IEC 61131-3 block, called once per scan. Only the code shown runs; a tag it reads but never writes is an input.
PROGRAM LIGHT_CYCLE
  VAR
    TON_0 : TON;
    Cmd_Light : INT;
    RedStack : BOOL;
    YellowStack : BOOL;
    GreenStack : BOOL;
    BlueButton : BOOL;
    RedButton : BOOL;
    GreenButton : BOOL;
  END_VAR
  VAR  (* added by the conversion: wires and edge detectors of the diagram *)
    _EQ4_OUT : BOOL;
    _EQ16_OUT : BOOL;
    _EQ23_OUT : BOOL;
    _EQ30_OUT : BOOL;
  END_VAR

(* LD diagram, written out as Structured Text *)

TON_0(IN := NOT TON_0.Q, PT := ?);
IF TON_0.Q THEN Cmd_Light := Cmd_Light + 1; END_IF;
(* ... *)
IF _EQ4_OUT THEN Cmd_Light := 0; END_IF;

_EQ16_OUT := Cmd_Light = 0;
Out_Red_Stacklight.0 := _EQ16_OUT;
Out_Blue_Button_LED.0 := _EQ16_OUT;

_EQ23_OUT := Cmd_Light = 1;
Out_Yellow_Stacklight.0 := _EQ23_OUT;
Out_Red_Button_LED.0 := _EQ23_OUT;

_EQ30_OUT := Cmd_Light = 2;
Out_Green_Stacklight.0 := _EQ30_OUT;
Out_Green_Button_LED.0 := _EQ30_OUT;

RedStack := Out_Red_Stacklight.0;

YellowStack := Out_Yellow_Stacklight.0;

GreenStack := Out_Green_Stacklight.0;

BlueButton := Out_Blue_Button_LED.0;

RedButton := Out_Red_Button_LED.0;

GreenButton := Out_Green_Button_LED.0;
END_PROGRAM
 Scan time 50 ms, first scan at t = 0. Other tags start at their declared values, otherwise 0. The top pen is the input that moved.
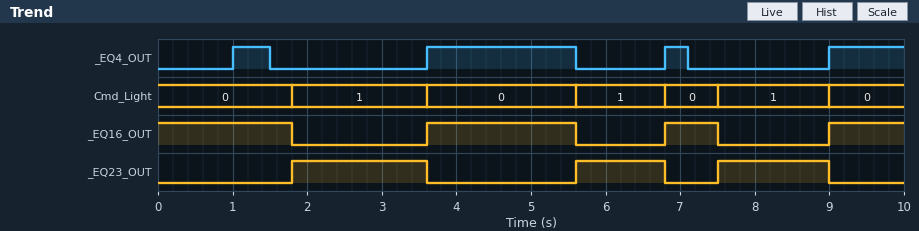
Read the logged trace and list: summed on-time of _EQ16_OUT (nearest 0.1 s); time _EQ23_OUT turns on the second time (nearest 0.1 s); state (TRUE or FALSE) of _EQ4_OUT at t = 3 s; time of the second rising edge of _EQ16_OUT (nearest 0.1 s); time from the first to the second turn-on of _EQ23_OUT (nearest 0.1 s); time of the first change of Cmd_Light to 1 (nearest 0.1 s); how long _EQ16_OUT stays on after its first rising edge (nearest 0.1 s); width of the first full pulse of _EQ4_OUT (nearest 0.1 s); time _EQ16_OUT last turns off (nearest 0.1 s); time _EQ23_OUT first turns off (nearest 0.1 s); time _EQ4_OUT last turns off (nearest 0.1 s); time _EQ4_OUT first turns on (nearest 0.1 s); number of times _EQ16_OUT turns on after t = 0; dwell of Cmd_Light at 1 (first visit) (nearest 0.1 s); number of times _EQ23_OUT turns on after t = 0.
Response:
5.5 s
5.6 s
FALSE
6.8 s
3.8 s
1.8 s
2.0 s
0.5 s
7.5 s
3.6 s
7.1 s
1.0 s
3
1.8 s
3
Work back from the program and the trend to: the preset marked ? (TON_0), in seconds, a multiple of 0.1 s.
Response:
1.8 s
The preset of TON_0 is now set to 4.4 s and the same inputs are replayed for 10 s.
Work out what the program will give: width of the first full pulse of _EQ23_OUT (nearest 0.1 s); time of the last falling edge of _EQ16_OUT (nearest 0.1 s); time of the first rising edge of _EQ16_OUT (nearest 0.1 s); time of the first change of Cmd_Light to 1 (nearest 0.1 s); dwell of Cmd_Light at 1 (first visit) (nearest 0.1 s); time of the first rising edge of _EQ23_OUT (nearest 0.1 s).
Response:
0.1 s
8.9 s
9.0 s
8.9 s
0.1 s
8.9 s
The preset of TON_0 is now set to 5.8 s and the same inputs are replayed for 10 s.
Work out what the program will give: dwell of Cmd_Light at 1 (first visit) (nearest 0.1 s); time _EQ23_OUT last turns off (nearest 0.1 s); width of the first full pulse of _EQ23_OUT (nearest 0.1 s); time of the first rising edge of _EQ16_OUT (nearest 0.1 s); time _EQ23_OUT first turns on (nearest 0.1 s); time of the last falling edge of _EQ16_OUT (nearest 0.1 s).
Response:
1.0 s
6.8 s
1.0 s
6.8 s
5.8 s
5.8 s
